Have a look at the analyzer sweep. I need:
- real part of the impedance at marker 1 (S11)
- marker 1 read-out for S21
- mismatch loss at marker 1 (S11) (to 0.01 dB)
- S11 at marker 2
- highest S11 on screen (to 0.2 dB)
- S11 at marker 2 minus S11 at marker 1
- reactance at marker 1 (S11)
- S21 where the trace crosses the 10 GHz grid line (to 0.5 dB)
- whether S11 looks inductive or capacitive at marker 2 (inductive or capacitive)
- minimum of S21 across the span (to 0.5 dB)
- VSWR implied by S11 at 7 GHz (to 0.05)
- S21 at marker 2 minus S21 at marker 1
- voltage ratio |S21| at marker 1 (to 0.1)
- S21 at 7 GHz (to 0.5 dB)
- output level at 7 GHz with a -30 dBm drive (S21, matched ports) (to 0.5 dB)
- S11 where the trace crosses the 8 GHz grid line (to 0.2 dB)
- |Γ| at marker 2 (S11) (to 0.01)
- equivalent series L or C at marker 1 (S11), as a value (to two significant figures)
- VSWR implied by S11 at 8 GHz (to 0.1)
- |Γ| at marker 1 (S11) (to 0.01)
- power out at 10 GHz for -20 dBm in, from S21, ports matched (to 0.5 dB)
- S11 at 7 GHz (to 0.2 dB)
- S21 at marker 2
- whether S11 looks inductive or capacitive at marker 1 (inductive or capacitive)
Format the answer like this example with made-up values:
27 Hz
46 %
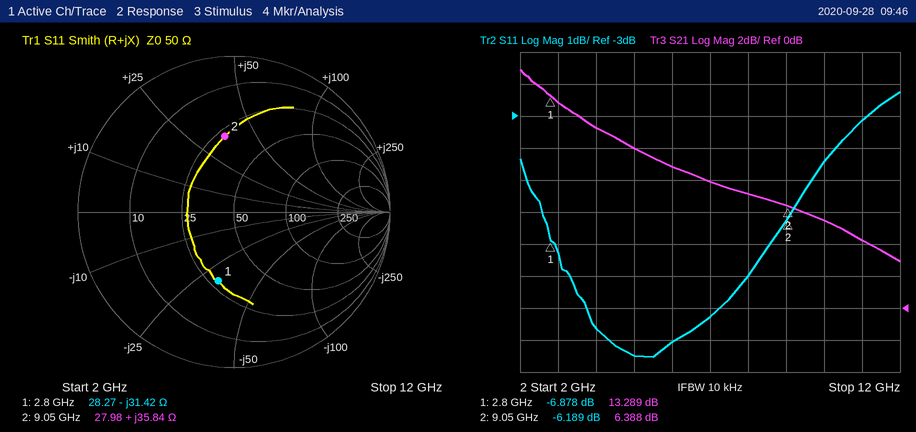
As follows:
28.27 Ω
13.289 dB
1.00 dB
-6.189 dB
-2.2 dB
0.689 dB
-31.42 Ω
5.5 dB
inductive
3.0 dB
2.05
-6.901 dB
4.6
8.0 dB
-22.0 dBm
-8.0 dB
0.49
1.8 pF
2.3
0.45
-14.5 dBm
-9.2 dB
6.388 dB
capacitive
